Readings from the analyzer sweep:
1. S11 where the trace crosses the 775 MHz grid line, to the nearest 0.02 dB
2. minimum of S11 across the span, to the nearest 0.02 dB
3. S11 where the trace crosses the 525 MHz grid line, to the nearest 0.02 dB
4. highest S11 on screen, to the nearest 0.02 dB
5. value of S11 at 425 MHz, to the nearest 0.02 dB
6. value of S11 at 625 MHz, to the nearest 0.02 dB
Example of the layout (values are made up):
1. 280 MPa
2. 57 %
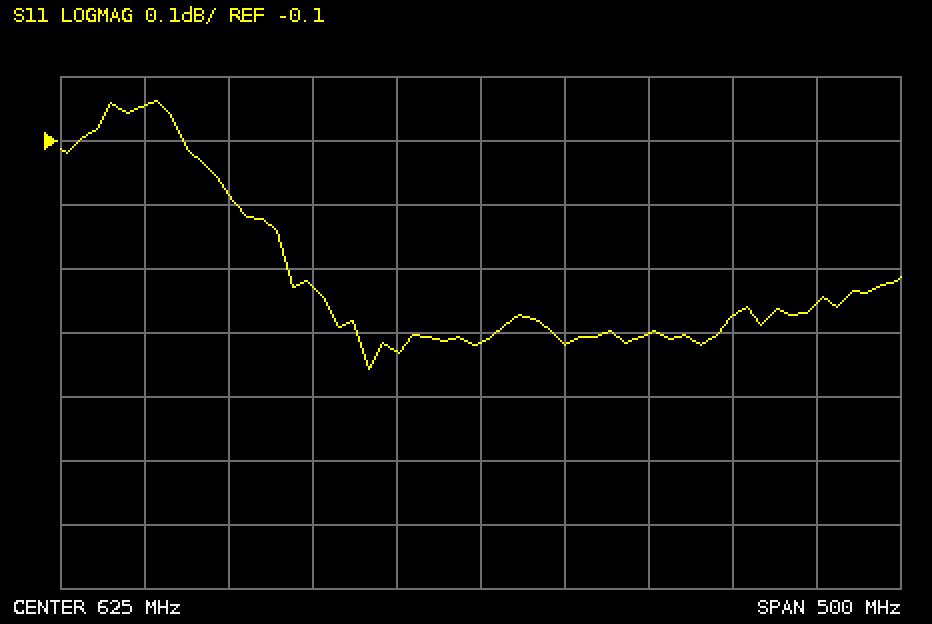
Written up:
1. -0.38 dB
2. -0.46 dB
3. -0.32 dB
4. -0.04 dB
5. -0.04 dB
6. -0.42 dB
